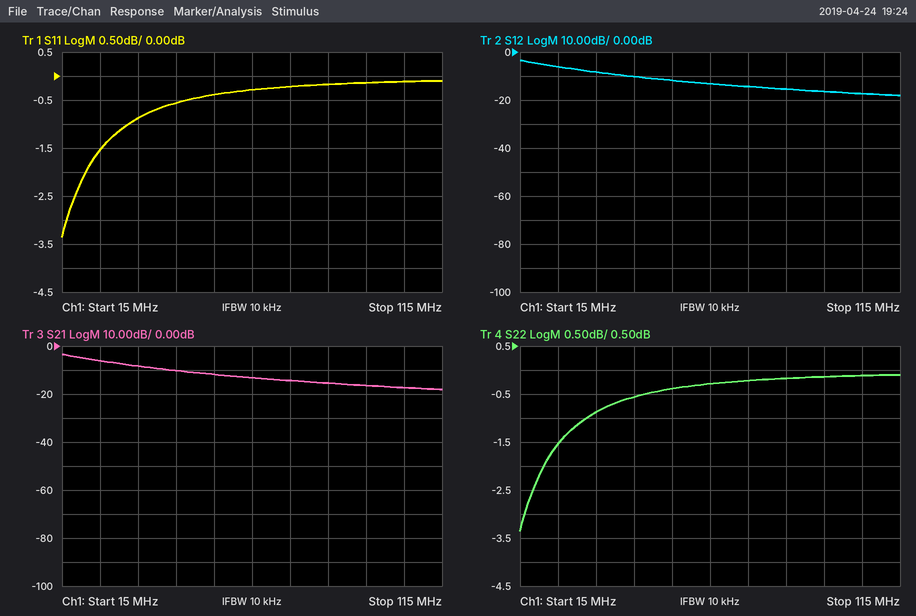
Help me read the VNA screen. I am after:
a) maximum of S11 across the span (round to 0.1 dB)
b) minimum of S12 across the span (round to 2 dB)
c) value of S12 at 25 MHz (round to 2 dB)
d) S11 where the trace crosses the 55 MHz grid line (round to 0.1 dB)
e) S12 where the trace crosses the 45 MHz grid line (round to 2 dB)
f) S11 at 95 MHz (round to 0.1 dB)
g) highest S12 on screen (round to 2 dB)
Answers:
-0.1 dB
-18 dB
-6 dB
-0.4 dB
-10 dB
-0.1 dB
-4 dB
